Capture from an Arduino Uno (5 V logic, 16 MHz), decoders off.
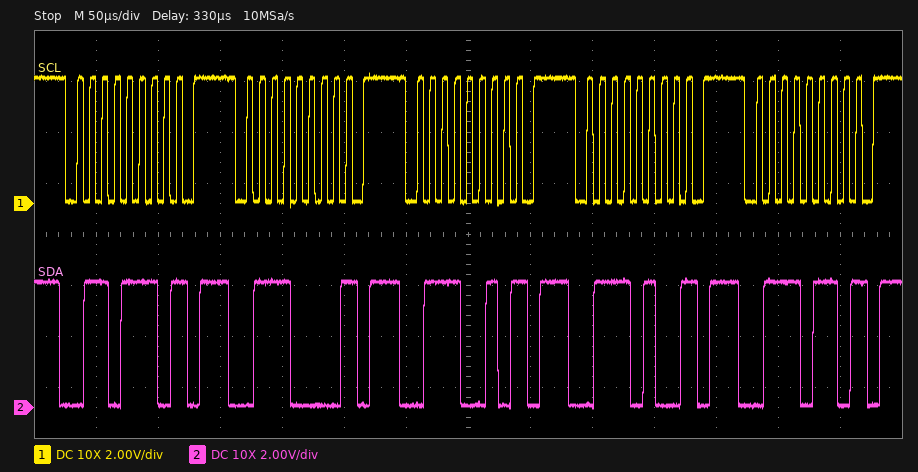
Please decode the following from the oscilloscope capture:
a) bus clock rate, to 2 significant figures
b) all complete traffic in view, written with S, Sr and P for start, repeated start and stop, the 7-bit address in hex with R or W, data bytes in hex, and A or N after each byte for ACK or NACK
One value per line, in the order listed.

100 kHz
S 37W N P S 38W N P S 39W N P S 3AW N P S 3BW N P
